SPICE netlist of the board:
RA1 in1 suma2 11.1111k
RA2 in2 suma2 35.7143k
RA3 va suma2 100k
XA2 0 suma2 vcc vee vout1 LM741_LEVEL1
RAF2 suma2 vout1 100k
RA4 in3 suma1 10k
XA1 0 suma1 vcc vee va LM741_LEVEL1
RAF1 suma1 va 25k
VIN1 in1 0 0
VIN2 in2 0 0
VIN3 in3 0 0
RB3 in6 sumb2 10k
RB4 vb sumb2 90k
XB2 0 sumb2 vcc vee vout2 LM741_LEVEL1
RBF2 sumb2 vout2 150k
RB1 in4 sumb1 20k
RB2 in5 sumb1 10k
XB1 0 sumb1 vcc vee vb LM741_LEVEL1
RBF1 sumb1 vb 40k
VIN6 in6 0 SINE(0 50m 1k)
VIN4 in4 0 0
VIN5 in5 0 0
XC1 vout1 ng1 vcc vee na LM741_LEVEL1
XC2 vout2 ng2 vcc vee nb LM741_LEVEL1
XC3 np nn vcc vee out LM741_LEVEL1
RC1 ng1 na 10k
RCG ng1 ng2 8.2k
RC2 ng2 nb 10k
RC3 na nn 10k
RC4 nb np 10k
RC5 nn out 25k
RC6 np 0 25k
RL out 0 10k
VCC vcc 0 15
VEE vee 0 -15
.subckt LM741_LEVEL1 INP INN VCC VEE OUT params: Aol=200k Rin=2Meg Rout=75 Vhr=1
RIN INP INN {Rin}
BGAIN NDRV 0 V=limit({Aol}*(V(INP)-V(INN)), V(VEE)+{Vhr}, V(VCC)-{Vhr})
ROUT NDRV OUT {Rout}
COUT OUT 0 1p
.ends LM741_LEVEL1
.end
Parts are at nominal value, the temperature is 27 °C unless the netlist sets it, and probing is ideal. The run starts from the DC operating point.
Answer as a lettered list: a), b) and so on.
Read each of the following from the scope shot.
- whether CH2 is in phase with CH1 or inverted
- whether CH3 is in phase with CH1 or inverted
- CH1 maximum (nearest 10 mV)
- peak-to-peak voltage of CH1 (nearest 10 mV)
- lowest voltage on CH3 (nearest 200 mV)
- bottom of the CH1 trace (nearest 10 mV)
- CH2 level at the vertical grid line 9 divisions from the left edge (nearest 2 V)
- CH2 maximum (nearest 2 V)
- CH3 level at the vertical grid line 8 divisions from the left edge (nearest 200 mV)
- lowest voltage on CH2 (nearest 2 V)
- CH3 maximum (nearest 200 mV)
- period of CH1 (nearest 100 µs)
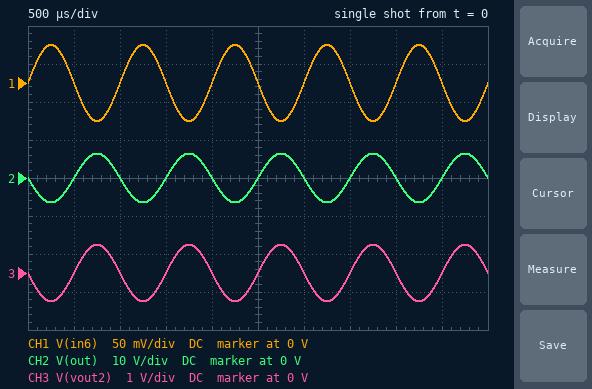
a) inverted
b) inverted
c) 50 mV
d) 100 mV
e) -800 mV
f) -50 mV
g) 0 V
h) 6 V
i) 0 V
j) -6 V
k) 800 mV
l) 1.0 ms
